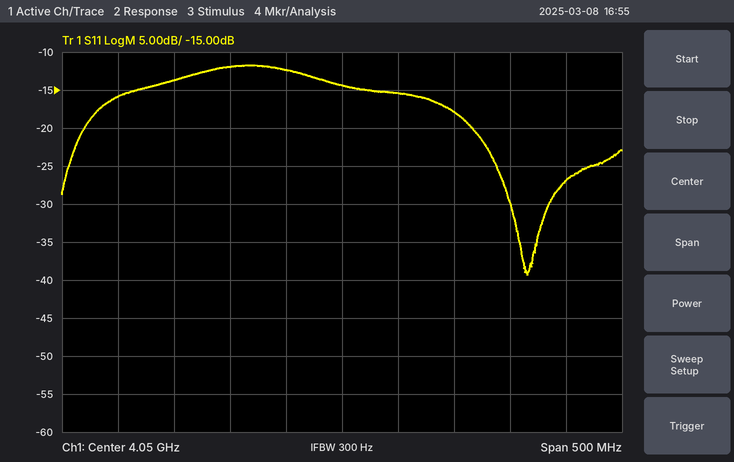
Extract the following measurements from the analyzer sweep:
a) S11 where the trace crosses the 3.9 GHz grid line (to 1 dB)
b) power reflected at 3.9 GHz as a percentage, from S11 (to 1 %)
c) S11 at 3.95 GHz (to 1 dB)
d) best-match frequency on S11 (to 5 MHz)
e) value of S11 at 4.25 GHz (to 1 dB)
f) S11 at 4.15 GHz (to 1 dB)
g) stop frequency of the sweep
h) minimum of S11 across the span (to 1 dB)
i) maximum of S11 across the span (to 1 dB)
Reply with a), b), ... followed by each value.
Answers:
a) -14 dB
b) 4 %
c) -12 dB
d) 4.215 GHz
e) -27 dB
f) -18 dB
g) 4.3 GHz
h) -39 dB
i) -12 dB
